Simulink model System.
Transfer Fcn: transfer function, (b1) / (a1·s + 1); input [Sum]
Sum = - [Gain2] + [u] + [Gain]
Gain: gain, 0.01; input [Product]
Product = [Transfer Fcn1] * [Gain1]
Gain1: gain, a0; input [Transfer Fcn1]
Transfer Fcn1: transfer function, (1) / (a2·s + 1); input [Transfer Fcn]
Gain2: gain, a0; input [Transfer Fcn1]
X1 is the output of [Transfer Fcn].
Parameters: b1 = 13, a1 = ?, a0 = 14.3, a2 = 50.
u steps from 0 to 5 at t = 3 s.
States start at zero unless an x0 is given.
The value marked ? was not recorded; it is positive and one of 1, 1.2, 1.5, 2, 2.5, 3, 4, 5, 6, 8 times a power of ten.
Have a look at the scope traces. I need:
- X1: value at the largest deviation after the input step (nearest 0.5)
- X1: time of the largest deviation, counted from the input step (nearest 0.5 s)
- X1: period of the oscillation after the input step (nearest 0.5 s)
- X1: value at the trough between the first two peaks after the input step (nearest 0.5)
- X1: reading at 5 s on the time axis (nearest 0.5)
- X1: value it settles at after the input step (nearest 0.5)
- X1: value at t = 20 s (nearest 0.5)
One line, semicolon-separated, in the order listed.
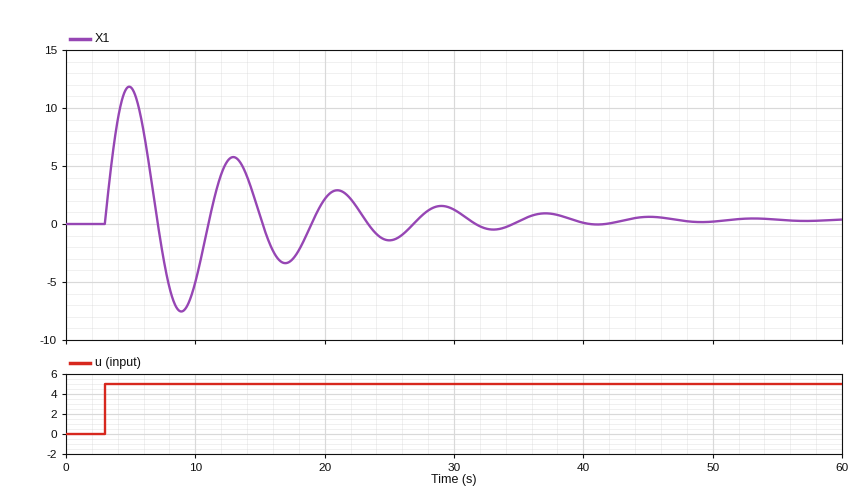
12.0; 2.0 s; 8.0 s; -7.5; 12.0; 0.5; 2.0
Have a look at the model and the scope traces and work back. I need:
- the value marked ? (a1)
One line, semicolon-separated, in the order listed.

6
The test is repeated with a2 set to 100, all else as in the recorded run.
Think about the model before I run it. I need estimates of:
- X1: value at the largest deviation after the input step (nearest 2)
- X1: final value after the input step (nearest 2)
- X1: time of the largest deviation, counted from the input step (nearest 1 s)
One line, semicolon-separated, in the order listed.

16; 0; 3 s
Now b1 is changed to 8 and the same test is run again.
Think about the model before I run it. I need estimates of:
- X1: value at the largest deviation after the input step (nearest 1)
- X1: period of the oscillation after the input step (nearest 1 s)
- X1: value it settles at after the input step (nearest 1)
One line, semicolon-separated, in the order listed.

9; 10 s; 0
